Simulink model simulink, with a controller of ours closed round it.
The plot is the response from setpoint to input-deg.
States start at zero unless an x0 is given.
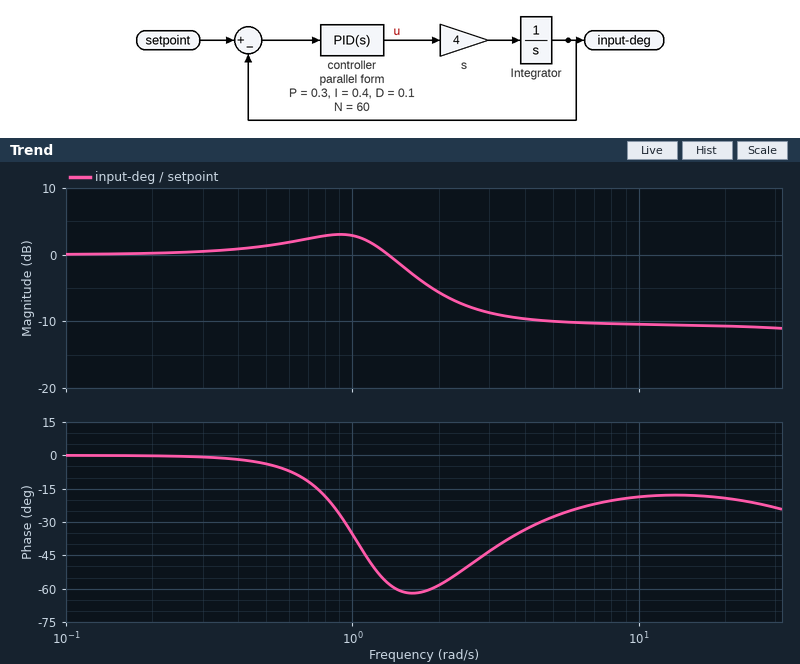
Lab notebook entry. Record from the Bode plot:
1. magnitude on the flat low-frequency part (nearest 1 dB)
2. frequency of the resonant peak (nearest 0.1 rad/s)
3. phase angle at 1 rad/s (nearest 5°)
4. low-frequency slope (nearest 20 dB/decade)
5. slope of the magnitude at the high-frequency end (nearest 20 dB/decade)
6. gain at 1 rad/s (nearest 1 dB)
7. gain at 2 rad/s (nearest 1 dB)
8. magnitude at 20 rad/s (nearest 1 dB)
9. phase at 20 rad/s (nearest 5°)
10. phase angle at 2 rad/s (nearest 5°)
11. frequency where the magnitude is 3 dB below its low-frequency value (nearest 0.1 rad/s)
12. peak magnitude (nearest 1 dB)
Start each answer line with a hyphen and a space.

- 0 dB
- 0.9 rad/s
- -35°
- 0 dB/decade
- 0 dB/decade
- 3 dB
- -6 dB
- -11 dB
- -20°
- -60°
- 1.6 rad/s
- 3 dB
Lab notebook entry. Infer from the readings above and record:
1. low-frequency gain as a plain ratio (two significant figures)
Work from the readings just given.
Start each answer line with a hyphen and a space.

- 1.0
